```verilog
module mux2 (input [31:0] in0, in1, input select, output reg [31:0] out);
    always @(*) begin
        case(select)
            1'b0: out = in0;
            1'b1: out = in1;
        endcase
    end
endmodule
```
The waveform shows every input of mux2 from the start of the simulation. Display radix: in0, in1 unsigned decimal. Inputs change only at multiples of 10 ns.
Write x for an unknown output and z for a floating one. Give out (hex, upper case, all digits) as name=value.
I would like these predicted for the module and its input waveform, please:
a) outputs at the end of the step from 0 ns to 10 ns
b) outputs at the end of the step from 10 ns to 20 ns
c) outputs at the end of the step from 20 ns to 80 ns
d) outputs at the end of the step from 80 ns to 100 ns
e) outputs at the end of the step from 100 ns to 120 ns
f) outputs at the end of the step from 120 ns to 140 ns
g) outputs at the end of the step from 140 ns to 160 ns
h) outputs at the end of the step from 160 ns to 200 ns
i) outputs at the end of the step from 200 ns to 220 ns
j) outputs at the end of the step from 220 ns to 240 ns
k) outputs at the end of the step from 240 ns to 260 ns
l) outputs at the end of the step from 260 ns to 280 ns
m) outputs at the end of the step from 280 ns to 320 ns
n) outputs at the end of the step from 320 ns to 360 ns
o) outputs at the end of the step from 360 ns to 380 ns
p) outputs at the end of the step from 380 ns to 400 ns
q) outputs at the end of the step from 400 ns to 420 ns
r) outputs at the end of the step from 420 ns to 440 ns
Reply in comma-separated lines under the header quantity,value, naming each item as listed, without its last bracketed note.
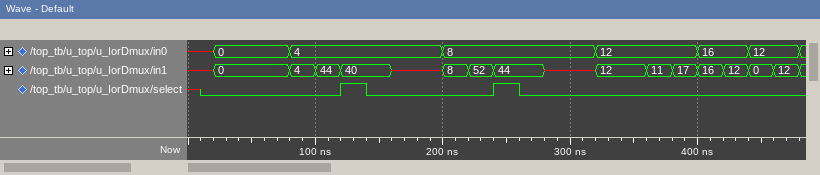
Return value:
quantity,value
outputs at the end of the step from 0 ns to 10 ns,out=x
outputs at the end of the step from 10 ns to 20 ns,out=x
outputs at the end of the step from 20 ns to 80 ns,out=00000000
outputs at the end of the step from 80 ns to 100 ns,out=00000004
outputs at the end of the step from 100 ns to 120 ns,out=00000004
outputs at the end of the step from 120 ns to 140 ns,out=00000028
outputs at the end of the step from 140 ns to 160 ns,out=00000004
outputs at the end of the step from 160 ns to 200 ns,out=00000004
outputs at the end of the step from 200 ns to 220 ns,out=00000008
outputs at the end of the step from 220 ns to 240 ns,out=00000008
outputs at the end of the step from 240 ns to 260 ns,out=0000002C
outputs at the end of the step from 260 ns to 280 ns,out=00000008
outputs at the end of the step from 280 ns to 320 ns,out=00000008
outputs at the end of the step from 320 ns to 360 ns,out=0000000C
outputs at the end of the step from 360 ns to 380 ns,out=0000000C
outputs at the end of the step from 380 ns to 400 ns,out=0000000C
outputs at the end of the step from 400 ns to 420 ns,out=00000010
outputs at the end of the step from 420 ns to 440 ns,out=00000010
